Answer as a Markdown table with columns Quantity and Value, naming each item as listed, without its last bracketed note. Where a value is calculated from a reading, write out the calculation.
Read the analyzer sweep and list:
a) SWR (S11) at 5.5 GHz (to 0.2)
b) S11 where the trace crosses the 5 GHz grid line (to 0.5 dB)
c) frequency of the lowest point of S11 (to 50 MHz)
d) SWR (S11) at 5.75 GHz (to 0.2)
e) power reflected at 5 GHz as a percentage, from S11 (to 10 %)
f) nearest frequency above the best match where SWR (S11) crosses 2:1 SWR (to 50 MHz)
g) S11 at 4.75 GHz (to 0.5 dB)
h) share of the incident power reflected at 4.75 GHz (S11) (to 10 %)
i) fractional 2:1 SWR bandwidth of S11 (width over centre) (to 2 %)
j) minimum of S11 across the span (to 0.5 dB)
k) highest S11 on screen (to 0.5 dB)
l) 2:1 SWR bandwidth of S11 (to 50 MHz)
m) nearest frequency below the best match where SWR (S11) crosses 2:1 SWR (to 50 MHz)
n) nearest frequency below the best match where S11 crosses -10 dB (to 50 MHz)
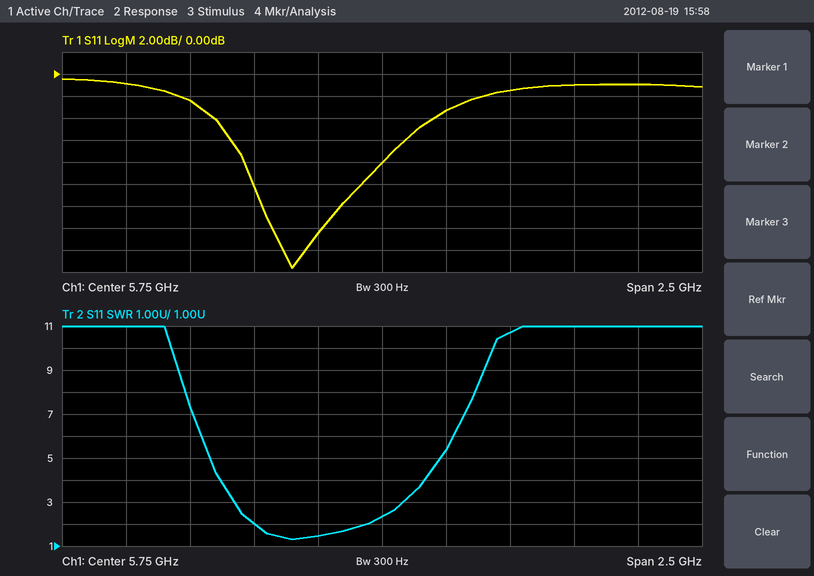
| Quantity | Value |
|---|---|
| SWR (S11) at 5.5 GHz | 1.4 |
| S11 where the trace crosses the 5 GHz grid line | -2.5 dB |
| frequency of the lowest point of S11 | 5.40 GHz |
| SWR (S11) at 5.75 GHz | 2.4 |
| power reflected at 5 GHz as a percentage, from S11 | 10^(-2.5/10) ≈ 56.2 %, so 60 % to the nearest 10 % |
| nearest frequency above the best match where SWR (S11) crosses 2:1 SWR | 5.70 GHz |
| S11 at 4.75 GHz | -1.0 dB |
| share of the incident power reflected at 4.75 GHz (S11) | 10^(-1/10) ≈ 79.4 %, so 80 % to the nearest 10 % |
| fractional 2:1 SWR bandwidth of S11 (width over centre) | 450 MHz / 5.475 GHz ≈ 8 % |
| minimum of S11 across the span | -17.5 dB |
| highest S11 on screen | -0.5 dB |
| 2:1 SWR bandwidth of S11 | 5.70 GHz − 5.25 GHz = 450 MHz |
| nearest frequency below the best match where SWR (S11) crosses 2:1 SWR | 5.25 GHz |
| nearest frequency below the best match where S11 crosses -10 dB | 5.25 GHz |
